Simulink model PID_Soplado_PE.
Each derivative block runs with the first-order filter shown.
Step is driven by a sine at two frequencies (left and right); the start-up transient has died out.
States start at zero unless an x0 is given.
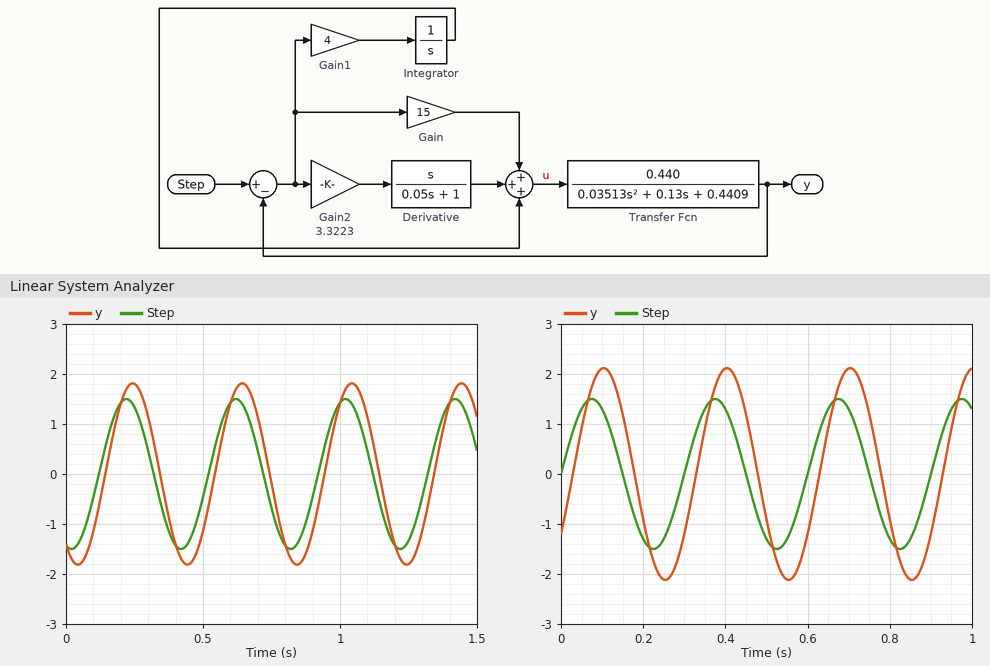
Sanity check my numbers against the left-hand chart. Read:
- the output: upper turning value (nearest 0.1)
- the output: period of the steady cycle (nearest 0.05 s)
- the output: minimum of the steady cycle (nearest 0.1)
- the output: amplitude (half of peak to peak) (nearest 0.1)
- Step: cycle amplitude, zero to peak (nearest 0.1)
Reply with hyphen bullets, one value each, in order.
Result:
- 1.8
- 0.40 s
- -1.8
- 1.8
- 1.5
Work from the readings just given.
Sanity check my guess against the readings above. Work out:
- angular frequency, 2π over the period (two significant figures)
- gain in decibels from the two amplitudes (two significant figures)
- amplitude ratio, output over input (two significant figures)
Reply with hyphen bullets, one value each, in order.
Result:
- 16 rad/s
- 1.6 dB
- 1.2
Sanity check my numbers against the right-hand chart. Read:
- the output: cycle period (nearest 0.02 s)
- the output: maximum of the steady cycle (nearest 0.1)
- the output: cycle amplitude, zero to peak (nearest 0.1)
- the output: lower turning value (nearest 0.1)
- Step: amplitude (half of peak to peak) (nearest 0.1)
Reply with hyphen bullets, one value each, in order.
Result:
- 0.30 s
- 2.1
- 2.1
- -2.1
- 1.5
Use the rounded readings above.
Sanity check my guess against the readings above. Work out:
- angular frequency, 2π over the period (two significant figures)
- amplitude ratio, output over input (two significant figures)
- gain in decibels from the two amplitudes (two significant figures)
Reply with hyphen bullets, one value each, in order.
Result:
- 21 rad/s
- 1.4
- 2.9 dB
